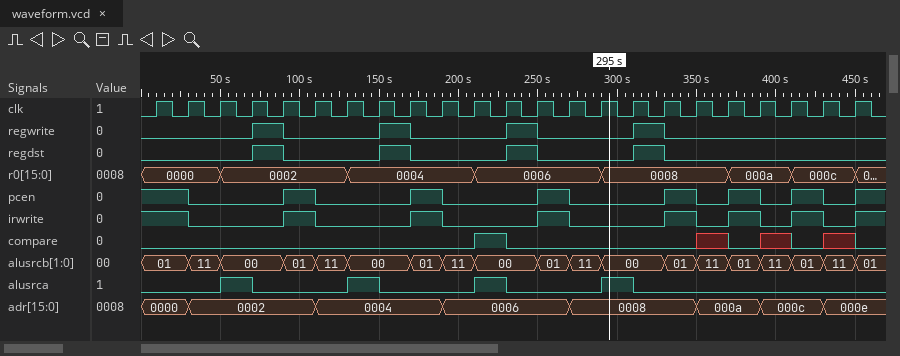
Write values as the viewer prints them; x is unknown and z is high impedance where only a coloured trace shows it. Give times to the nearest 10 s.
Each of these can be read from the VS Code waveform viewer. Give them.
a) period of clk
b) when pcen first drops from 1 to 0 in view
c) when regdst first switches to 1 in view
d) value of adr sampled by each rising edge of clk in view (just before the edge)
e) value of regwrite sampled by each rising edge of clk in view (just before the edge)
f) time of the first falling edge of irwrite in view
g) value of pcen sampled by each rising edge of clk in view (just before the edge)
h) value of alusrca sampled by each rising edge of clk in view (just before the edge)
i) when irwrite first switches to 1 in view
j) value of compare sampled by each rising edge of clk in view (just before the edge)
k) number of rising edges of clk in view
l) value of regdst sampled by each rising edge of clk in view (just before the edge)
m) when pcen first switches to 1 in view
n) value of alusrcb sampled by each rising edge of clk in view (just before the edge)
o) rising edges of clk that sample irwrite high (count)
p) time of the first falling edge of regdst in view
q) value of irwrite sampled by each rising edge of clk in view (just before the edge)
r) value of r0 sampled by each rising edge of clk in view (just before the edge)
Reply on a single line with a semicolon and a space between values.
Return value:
20 s; 30 s; 70 s; 0000, 0000, 0002, 0002, 0002, 0002, 0004, 0004, 0004, 0004, 0006, 0006, 0006, 0006, 0008, 0008, 0008, 0008, 000a, 000a, 000c, 000c, 000e; 0 0 0 0 1 0 0 0 1 0 0 0 1 0 0 0 1 0 0 0 0 0 0; 30 s; 1 1 0 0 0 1 0 0 0 1 0 0 0 1 0 0 0 1 0 1 0 1 0; 0 0 0 1 0 0 0 1 0 0 0 1 0 0 0 1 0 0 0 0 0 0 0; 90 s; 0 0 0 0 0 0 0 0 0 0 0 1 0 0 0 0 0 0 x 0 x 0 x; 23; 0 0 0 0 1 0 0 0 1 0 0 0 1 0 0 0 1 0 0 0 0 0 0; 90 s; 01, 01, 11, 00, 00, 01, 11, 00, 00, 01, 11, 00, 00, 01, 11, 00, 00, 01, 11, 01, 11, 01, 11; 8; 90 s; 1 1 0 0 0 1 0 0 0 1 0 0 0 1 0 0 0 1 0 1 0 1 0; 0000, 0000, 0000, 0002, 0002, 0002, 0002, 0004, 0004, 0004, 0004, 0006, 0006, 0006, 0006, 0008, 0008, 0008, 0008, 000a, 000a, 000c, 000c
